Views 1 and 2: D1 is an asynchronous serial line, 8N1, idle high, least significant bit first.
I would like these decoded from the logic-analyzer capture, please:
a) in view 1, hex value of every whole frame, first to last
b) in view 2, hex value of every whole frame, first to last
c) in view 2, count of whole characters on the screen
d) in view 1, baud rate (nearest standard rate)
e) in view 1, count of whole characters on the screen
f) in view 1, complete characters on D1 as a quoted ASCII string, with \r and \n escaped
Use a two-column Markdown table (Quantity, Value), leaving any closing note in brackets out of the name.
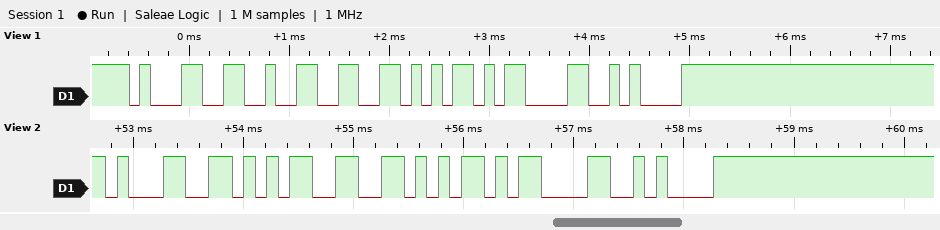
| Quantity | Value |
|---|---|
| in view 1, hex value of every whole frame, first to last | 0x31 0x32 0x56 0x0D 0x0A |
| in view 2, hex value of every whole frame, first to last | 31 35 56 0D 0A |
| in view 2, count of whole characters on the screen | 5 |
| in view 1, baud rate | 9600 baud |
| in view 1, count of whole characters on the screen | 5 |
| in view 1, complete characters on D1 as a quoted ASCII string, with \r and \n escaped | "12V\r\n" |
